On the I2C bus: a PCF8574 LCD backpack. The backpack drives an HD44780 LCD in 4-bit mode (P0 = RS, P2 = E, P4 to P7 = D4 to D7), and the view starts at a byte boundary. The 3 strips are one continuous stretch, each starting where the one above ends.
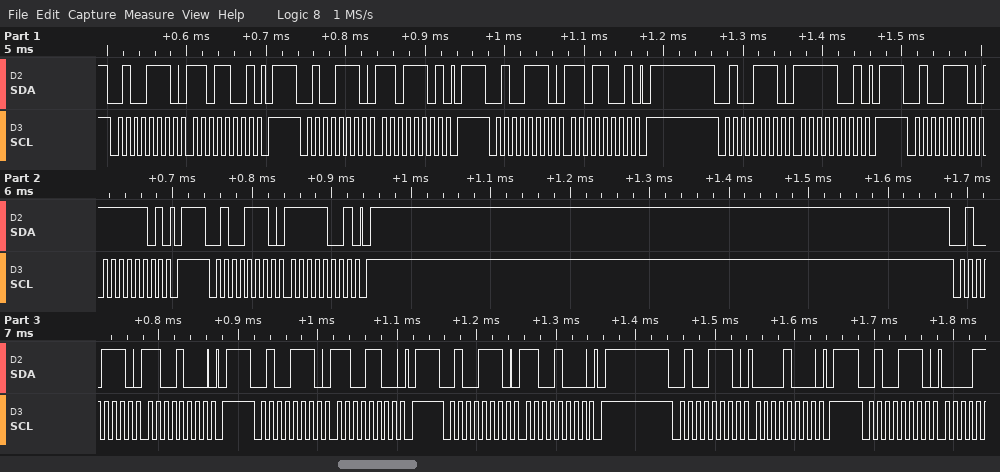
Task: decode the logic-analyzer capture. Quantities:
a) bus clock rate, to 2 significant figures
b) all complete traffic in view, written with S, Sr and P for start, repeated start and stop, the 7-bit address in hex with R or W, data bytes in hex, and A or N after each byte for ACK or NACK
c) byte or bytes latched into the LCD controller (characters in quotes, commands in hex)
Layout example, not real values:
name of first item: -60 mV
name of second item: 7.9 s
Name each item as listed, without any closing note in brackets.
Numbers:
bus clock rate, to 2 significant figures: 100 kHz
all complete traffic in view, written with S, Sr and P for start, repeated start and stop, the 7-bit address in hex with R or W, data bytes in hex, and A or N after each byte for ACK or NACK: S 27W A D9 A P S 27W A DD A P S 27W A D9 A P S 27W A F9 A P S 27W A FD A P S 27W A F9 A P S 27W A C8 A P S 27W A CC A P S 27W A C8 A P S 27W A 08 A P S 27W A
byte or bytes latched into the LCD controller: data 0xDF
